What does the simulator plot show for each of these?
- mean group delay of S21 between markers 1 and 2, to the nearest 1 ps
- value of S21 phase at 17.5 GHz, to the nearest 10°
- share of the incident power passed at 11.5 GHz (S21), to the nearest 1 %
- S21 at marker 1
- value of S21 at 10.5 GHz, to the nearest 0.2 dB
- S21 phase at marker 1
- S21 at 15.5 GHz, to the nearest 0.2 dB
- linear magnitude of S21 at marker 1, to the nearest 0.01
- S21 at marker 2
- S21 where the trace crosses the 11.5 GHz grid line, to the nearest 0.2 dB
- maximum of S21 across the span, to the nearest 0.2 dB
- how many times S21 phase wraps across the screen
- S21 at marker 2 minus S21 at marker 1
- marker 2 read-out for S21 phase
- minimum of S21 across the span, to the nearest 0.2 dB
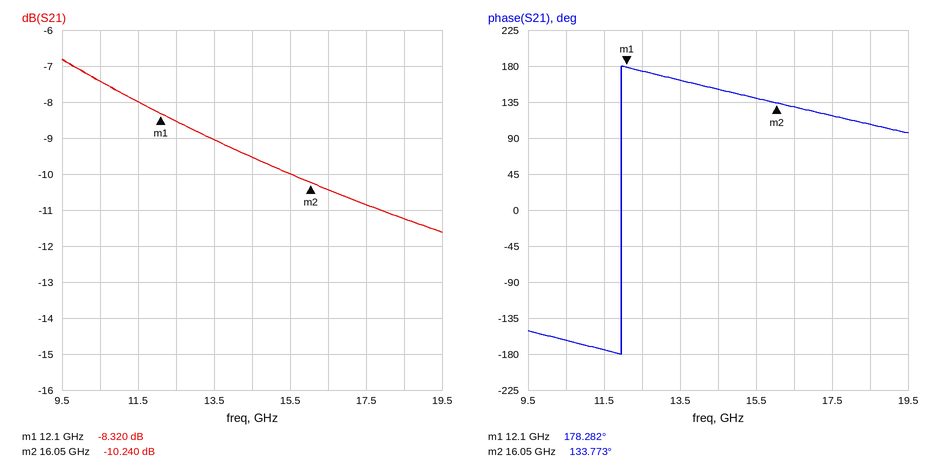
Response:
31 ps
120°
16 %
-8.320 dB
-7.4 dB
178.282°
-10.0 dB
0.38
-10.240 dB
-8.0 dB
-6.8 dB
1
-1.920 dB
133.773°
-11.6 dB
